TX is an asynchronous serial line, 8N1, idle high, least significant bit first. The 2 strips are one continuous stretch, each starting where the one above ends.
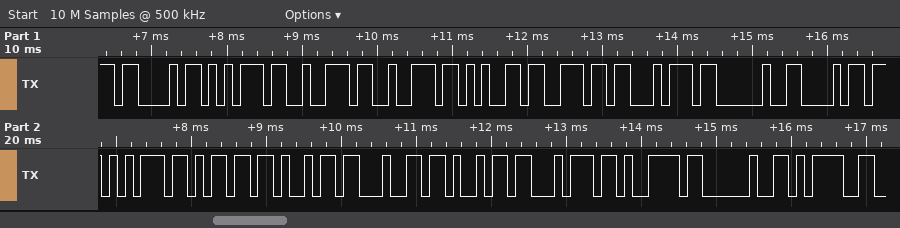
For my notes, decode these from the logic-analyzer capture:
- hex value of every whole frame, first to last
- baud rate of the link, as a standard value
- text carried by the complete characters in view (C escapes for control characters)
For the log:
43 75 72 72 65 6E 74 20 68 75 6D 69 64 69 74 79 20 3D
9600 baud
"Current humidity ="
